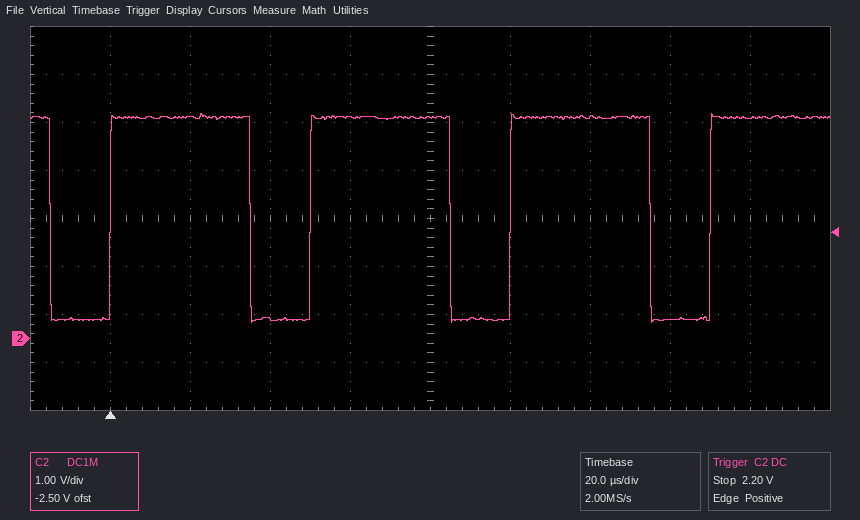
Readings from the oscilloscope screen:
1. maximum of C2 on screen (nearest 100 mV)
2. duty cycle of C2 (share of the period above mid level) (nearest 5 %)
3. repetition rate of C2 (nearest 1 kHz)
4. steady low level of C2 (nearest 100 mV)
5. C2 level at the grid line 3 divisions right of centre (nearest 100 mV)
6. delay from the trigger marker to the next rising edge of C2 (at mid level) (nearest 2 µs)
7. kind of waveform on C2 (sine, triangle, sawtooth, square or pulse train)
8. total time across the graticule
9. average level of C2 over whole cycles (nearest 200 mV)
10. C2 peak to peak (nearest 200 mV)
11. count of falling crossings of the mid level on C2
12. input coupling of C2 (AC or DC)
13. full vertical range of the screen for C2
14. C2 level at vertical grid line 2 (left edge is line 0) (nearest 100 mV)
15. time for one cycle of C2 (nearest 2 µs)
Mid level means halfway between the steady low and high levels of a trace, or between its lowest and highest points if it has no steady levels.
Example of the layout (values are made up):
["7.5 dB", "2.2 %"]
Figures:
["4.7 V", "70 %", "20 kHz", "400 mV", "400 mV", "50 µs", "pulse train", "200 µs", "3.4 V", "4.4 V", "4", "DC", "8 V", "4.6 V", "50 µs"]
